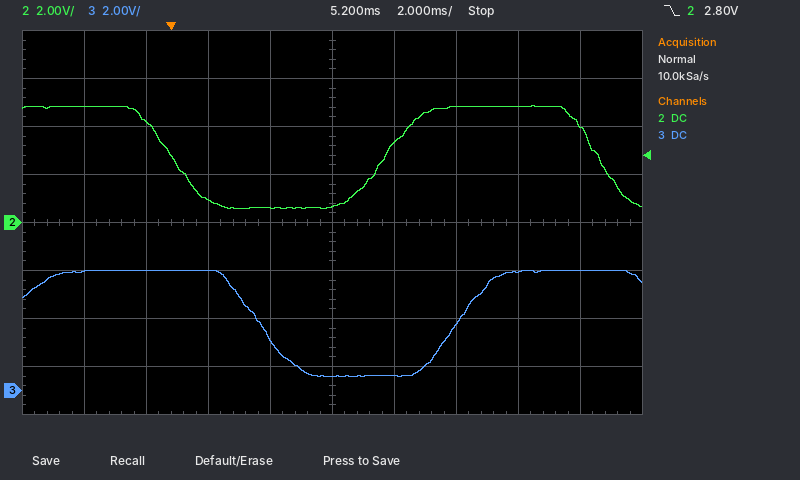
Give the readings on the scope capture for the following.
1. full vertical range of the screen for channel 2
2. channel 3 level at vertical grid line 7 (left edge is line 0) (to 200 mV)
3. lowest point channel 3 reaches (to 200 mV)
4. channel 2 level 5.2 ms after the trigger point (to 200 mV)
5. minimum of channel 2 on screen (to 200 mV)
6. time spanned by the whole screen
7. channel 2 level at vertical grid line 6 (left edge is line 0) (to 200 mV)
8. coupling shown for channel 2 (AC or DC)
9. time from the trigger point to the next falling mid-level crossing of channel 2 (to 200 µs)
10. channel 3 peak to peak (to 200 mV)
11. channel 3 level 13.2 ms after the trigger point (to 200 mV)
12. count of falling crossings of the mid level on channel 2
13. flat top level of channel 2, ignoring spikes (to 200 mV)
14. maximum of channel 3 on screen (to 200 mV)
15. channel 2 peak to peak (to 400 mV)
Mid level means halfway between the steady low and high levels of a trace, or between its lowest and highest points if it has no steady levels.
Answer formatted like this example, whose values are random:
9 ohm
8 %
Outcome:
16 V
2.8 V
600 mV
600 mV
600 mV
20 ms
3.4 V
DC
13.8 ms
4.4 V
5.0 V
2
4.8 V
5.0 V
4.4 V
